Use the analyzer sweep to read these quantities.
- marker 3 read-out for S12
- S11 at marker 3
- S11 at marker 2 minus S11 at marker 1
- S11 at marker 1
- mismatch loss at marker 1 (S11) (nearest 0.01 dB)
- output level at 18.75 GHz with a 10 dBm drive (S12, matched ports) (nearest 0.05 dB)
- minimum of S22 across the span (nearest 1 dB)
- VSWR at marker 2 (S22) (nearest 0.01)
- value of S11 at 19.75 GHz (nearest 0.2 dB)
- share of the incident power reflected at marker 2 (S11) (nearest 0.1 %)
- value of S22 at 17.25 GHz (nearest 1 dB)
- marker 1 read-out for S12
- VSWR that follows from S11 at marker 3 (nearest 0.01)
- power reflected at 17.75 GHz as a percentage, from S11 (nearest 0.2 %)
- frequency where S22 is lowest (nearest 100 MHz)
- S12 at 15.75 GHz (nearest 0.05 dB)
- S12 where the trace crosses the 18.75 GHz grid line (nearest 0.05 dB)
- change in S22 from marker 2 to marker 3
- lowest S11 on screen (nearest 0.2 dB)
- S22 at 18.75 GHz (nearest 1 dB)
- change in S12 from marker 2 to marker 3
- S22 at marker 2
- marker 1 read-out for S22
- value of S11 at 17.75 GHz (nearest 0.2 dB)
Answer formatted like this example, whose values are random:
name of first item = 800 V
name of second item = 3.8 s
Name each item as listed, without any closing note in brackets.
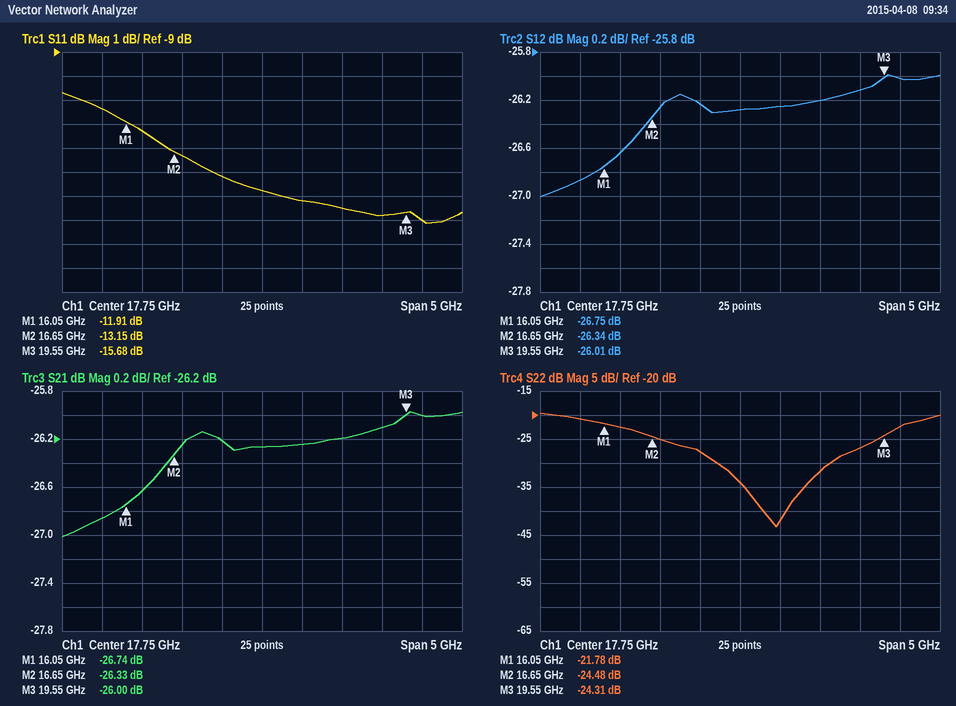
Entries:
marker 3 read-out for S12 = -26.01 dB
S11 at marker 3 = -15.68 dB
S11 at marker 2 minus S11 at marker 1 = -1.24 dB
S11 at marker 1 = -11.91 dB
mismatch loss at marker 1 (S11) = 0.29 dB
output level at 18.75 GHz with a 10 dBm drive (S12, matched ports) = -16.20 dBm
minimum of S22 across the span = -43 dB
VSWR at marker 2 (S22) = 1.13
value of S11 at 19.75 GHz = -16.0 dB
share of the incident power reflected at marker 2 (S11) = 4.8 %
value of S22 at 17.25 GHz = -28 dB
marker 1 read-out for S12 = -26.75 dB
VSWR that follows from S11 at marker 3 = 1.39
power reflected at 17.75 GHz as a percentage, from S11 = 3.4 %
frequency where S22 is lowest = 18.2 GHz
S12 at 15.75 GHz = -26.85 dB
S12 where the trace crosses the 18.75 GHz grid line = -26.20 dB
change in S22 from marker 2 to marker 3 = 0.17 dB
lowest S11 on screen = -16.2 dB
S22 at 18.75 GHz = -32 dB
change in S12 from marker 2 to marker 3 = 0.33 dB
S22 at marker 2 = -24.48 dB
marker 1 read-out for S22 = -21.78 dB
value of S11 at 17.75 GHz = -14.8 dB
